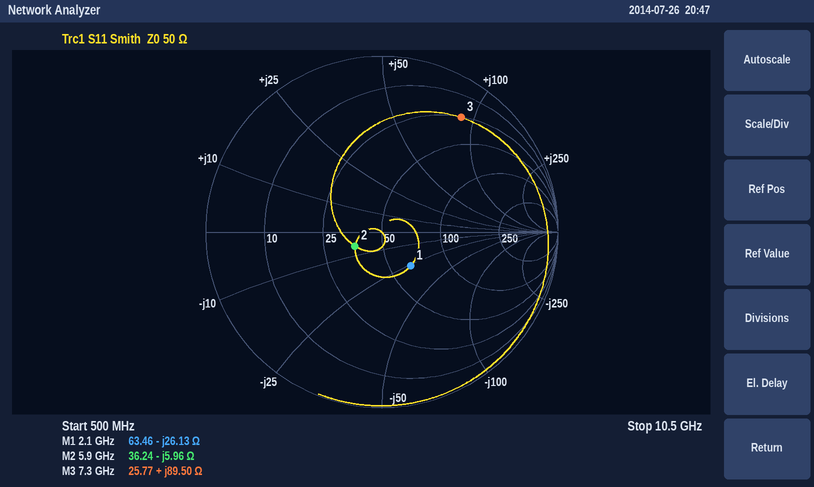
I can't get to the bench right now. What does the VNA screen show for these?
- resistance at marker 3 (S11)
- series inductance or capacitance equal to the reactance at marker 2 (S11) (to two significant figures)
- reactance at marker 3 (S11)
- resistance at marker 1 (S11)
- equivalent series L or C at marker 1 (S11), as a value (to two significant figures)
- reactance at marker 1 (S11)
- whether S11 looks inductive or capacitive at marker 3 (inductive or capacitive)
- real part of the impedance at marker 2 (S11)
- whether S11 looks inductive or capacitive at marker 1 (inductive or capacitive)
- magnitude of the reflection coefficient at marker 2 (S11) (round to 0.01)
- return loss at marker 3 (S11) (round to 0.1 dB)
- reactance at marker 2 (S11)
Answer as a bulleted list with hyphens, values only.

- 25.77 Ω
- 4.5 pF
- +89.50 Ω
- 63.46 Ω
- 2.9 pF
- -26.13 Ω
- inductive
- 36.24 Ω
- capacitive
- 0.17
- 2.0 dB
- -5.96 Ω
